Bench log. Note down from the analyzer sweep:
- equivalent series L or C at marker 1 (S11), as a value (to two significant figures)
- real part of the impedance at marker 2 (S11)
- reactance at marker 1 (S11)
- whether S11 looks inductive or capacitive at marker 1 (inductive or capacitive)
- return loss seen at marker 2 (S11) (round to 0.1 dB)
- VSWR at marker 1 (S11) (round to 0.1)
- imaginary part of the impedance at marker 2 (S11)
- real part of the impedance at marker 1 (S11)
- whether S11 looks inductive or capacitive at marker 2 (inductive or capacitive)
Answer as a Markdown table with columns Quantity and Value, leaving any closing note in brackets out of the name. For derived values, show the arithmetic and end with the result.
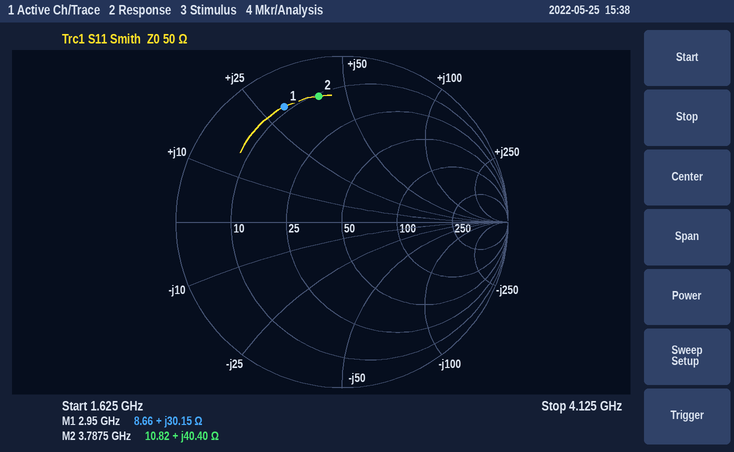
| Quantity | Value |
|---|---|
| equivalent series L or C at marker 1 (S11), as a value | L = 30.15 Ω/(2π × 2.95 GHz) ≈ 1.6 nH |
| real part of the impedance at marker 2 | 10.82 Ω |
| reactance at marker 1 | +30.15 Ω |
| whether S11 looks inductive or capacitive at marker 1 | inductive |
| return loss seen at marker 2 (S11) | 2.3 dB |
| VSWR at marker 1 (S11) | 7.9 |
| imaginary part of the impedance at marker 2 | +40.40 Ω |
| real part of the impedance at marker 1 | 8.66 Ω |
| whether S11 looks inductive or capacitive at marker 2 | inductive |
